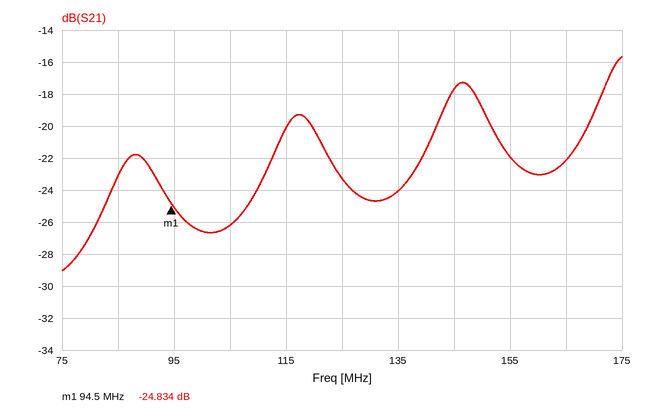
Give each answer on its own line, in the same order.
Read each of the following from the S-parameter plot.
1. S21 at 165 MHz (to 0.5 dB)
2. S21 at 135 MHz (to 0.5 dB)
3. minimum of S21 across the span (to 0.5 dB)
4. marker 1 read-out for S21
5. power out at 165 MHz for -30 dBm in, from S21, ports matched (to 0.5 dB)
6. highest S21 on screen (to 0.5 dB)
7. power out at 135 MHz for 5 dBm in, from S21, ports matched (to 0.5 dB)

-22.0 dB
-24.0 dB
-29.0 dB
-24.834 dB
-52.0 dBm
-15.5 dB
-19.0 dBm
